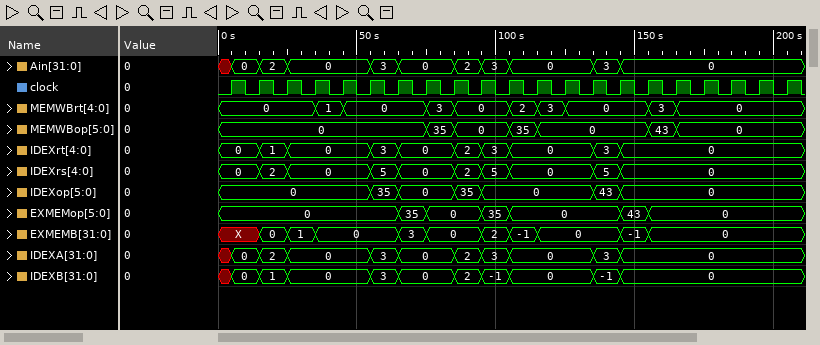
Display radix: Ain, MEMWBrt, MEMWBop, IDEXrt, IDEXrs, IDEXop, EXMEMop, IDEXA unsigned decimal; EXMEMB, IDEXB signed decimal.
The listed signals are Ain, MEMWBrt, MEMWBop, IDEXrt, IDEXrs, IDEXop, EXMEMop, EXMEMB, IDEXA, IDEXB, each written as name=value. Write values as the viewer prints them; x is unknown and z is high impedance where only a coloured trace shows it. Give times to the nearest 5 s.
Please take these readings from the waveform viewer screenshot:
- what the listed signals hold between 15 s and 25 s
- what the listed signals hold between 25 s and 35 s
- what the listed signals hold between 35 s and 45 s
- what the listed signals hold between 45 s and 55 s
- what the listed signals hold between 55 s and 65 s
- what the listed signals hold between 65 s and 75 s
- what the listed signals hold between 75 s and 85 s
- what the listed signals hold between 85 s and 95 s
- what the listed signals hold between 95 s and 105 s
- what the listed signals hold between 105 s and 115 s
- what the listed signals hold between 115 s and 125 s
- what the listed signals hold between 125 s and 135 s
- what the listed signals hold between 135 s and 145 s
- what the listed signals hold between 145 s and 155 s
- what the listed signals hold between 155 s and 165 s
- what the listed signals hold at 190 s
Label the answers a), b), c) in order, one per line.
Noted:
a) Ain=2, MEMWBrt=0, MEMWBop=0, IDEXrt=1, IDEXrs=2, IDEXop=0, EXMEMop=0, EXMEMB=0, IDEXA=2, IDEXB=1
b) Ain=0, MEMWBrt=0, MEMWBop=0, IDEXrt=0, IDEXrs=0, IDEXop=0, EXMEMop=0, EXMEMB=1, IDEXA=0, IDEXB=0
c) Ain=0, MEMWBrt=1, MEMWBop=0, IDEXrt=0, IDEXrs=0, IDEXop=0, EXMEMop=0, EXMEMB=0, IDEXA=0, IDEXB=0
d) Ain=0, MEMWBrt=0, MEMWBop=0, IDEXrt=0, IDEXrs=0, IDEXop=0, EXMEMop=0, EXMEMB=0, IDEXA=0, IDEXB=0
e) Ain=3, MEMWBrt=0, MEMWBop=0, IDEXrt=3, IDEXrs=5, IDEXop=35, EXMEMop=0, EXMEMB=0, IDEXA=3, IDEXB=3
f) Ain=0, MEMWBrt=0, MEMWBop=0, IDEXrt=0, IDEXrs=0, IDEXop=0, EXMEMop=35, EXMEMB=3, IDEXA=0, IDEXB=0
g) Ain=0, MEMWBrt=3, MEMWBop=35, IDEXrt=0, IDEXrs=0, IDEXop=0, EXMEMop=0, EXMEMB=0, IDEXA=0, IDEXB=0
h) Ain=2, MEMWBrt=0, MEMWBop=0, IDEXrt=2, IDEXrs=2, IDEXop=35, EXMEMop=0, EXMEMB=0, IDEXA=2, IDEXB=2
i) Ain=3, MEMWBrt=0, MEMWBop=0, IDEXrt=3, IDEXrs=5, IDEXop=0, EXMEMop=35, EXMEMB=2, IDEXA=3, IDEXB=-1
j) Ain=0, MEMWBrt=2, MEMWBop=35, IDEXrt=0, IDEXrs=0, IDEXop=0, EXMEMop=0, EXMEMB=-1, IDEXA=0, IDEXB=0
k) Ain=0, MEMWBrt=3, MEMWBop=0, IDEXrt=0, IDEXrs=0, IDEXop=0, EXMEMop=0, EXMEMB=0, IDEXA=0, IDEXB=0
l) Ain=0, MEMWBrt=0, MEMWBop=0, IDEXrt=0, IDEXrs=0, IDEXop=0, EXMEMop=0, EXMEMB=0, IDEXA=0, IDEXB=0
m) Ain=3, MEMWBrt=0, MEMWBop=0, IDEXrt=3, IDEXrs=5, IDEXop=43, EXMEMop=0, EXMEMB=0, IDEXA=3, IDEXB=-1
n) Ain=0, MEMWBrt=0, MEMWBop=0, IDEXrt=0, IDEXrs=0, IDEXop=0, EXMEMop=43, EXMEMB=-1, IDEXA=0, IDEXB=0
o) Ain=0, MEMWBrt=3, MEMWBop=43, IDEXrt=0, IDEXrs=0, IDEXop=0, EXMEMop=0, EXMEMB=0, IDEXA=0, IDEXB=0
p) Ain=0, MEMWBrt=0, MEMWBop=0, IDEXrt=0, IDEXrs=0, IDEXop=0, EXMEMop=0, EXMEMB=0, IDEXA=0, IDEXB=0
